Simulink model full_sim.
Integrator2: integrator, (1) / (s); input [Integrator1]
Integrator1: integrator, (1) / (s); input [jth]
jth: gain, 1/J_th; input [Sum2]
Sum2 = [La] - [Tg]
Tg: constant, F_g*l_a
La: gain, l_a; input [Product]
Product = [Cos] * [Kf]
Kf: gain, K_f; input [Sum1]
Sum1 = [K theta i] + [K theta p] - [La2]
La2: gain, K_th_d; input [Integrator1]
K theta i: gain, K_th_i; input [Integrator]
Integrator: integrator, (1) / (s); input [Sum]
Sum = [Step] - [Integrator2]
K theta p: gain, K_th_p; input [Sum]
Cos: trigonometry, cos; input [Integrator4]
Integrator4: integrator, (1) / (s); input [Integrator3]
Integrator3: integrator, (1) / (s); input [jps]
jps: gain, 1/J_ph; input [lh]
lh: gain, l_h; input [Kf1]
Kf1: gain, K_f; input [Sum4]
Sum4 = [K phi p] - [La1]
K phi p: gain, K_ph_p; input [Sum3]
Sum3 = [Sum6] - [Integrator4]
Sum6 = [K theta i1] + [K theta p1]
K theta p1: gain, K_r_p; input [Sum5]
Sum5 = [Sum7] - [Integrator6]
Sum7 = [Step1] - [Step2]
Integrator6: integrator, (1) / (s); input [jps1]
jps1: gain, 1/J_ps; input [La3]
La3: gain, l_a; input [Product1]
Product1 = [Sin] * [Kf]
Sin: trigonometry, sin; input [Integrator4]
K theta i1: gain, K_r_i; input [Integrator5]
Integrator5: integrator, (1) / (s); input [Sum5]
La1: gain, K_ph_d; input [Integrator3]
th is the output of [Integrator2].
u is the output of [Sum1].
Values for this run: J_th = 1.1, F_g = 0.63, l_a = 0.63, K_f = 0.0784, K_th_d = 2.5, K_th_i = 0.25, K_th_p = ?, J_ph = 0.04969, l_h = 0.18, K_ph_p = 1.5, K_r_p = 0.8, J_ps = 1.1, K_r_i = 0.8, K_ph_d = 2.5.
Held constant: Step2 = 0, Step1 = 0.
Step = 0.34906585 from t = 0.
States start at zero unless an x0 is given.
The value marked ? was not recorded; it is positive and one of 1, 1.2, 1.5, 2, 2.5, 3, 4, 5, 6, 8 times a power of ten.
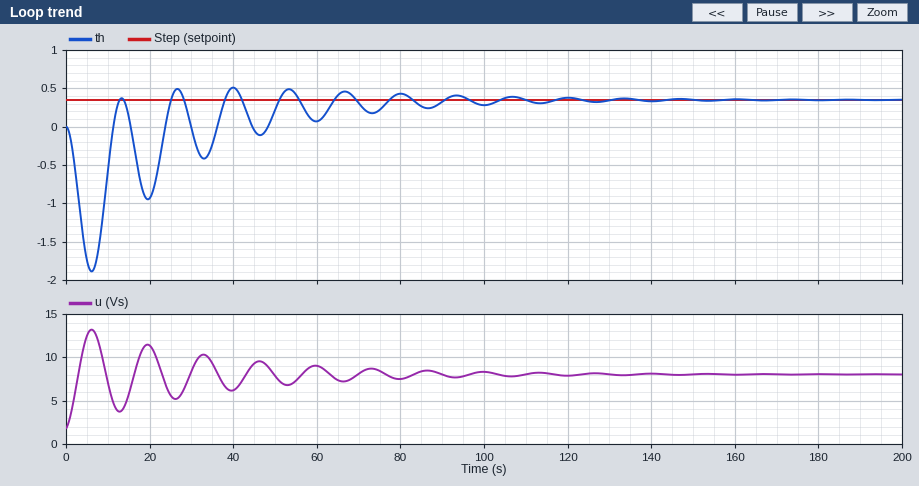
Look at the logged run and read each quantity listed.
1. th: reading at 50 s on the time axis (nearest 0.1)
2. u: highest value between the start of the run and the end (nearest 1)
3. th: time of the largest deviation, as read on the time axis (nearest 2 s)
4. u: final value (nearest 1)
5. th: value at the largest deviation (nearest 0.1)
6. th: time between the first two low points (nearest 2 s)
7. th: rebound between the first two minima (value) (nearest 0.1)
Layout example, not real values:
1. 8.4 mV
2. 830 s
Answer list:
1. 0.2
2. 13
3. 6 s
4. 8
5. -1.9
6. 14 s
7. 0.4
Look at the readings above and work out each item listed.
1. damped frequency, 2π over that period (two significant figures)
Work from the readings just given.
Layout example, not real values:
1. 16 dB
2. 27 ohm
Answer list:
1. 0.45 rad/s
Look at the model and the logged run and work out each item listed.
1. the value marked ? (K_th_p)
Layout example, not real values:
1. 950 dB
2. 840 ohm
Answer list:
1. 5
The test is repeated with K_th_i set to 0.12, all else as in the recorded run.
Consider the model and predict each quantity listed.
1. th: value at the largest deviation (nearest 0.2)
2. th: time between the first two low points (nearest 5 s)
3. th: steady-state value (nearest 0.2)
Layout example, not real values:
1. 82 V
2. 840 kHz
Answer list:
1. -2.0
2. 15 s
3. 0.4
